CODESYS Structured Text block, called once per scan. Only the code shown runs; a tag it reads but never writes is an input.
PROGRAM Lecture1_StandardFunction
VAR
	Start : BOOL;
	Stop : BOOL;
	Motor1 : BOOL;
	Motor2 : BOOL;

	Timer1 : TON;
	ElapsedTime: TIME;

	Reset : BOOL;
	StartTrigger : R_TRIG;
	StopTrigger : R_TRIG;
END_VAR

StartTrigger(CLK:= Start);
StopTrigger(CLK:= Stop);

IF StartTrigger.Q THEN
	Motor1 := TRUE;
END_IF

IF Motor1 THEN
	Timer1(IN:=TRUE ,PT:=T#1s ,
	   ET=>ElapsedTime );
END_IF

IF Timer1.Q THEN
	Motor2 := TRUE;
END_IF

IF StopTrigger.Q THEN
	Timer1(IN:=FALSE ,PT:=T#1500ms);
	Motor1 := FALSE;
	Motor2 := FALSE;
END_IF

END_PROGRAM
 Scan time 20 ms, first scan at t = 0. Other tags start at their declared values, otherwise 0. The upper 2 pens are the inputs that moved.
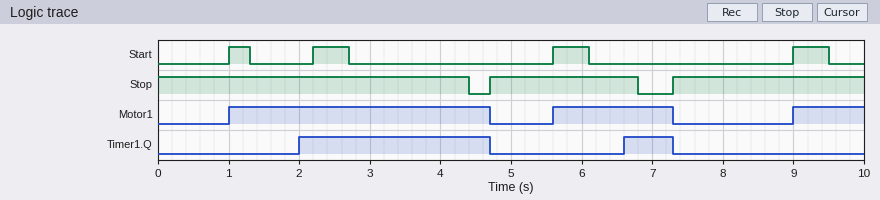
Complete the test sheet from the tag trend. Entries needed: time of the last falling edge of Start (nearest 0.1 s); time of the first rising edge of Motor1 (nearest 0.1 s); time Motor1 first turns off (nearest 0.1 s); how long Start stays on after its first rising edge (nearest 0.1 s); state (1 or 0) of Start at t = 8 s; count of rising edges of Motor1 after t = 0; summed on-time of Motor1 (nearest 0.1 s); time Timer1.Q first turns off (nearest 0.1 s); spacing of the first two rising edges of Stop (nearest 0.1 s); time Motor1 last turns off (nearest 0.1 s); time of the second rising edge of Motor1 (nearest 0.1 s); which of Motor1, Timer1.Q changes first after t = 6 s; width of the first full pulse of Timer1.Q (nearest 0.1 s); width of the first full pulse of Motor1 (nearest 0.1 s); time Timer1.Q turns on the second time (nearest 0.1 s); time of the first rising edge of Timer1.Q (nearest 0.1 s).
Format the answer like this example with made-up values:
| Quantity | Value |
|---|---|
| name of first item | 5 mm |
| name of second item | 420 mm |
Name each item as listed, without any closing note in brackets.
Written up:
| Quantity | Value |
|---|---|
| time of the last falling edge of Start | 9.5 s |
| time of the first rising edge of Motor1 | 1.0 s |
| time Motor1 first turns off | 4.7 s |
| how long Start stays on after its first rising edge | 0.3 s |
| state (1 or 0) of Start at t = 8 s | 0 |
| count of rising edges of Motor1 after t = 0 | 3 |
| summed on-time of Motor1 | 6.4 s |
| time Timer1.Q first turns off | 4.7 s |
| spacing of the first two rising edges of Stop | 2.6 s |
| time Motor1 last turns off | 7.3 s |
| time of the second rising edge of Motor1 | 5.6 s |
| which of Motor1, Timer1.Q changes first after t = 6 s | Timer1.Q |
| width of the first full pulse of Timer1.Q | 2.7 s |
| width of the first full pulse of Motor1 | 3.7 s |
| time Timer1.Q turns on the second time | 6.6 s |
| time of the first rising edge of Timer1.Q | 2.0 s |
